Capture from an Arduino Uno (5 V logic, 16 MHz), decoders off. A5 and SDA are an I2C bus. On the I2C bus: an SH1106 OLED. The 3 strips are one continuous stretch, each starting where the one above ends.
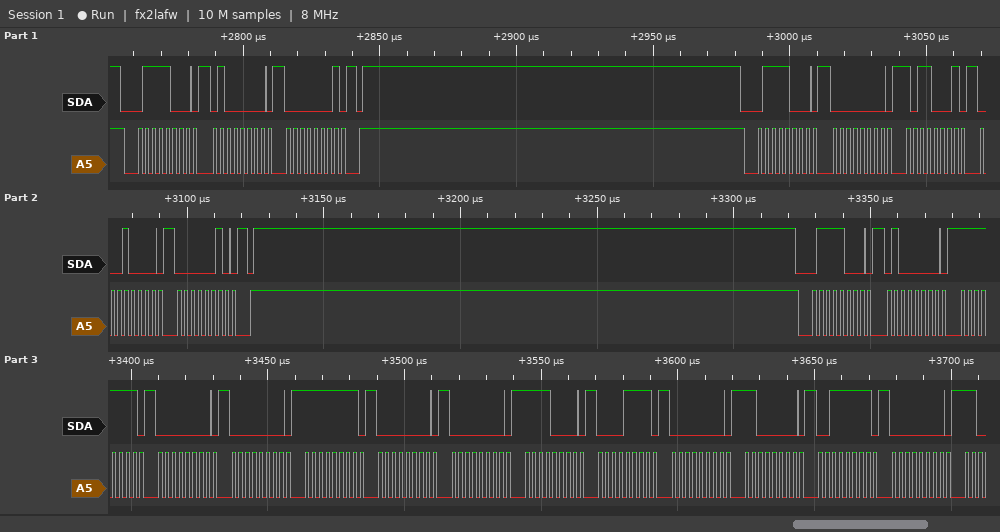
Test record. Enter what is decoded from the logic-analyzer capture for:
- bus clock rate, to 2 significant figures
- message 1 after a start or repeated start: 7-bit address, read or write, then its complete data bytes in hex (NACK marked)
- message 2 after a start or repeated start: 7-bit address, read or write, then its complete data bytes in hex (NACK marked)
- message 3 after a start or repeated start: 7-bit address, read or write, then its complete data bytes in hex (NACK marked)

400 kHz
0x3C write: 40 01
0x3C write: 00 B1 10 02
0x3C write: 40 FF 00 00 FF 00 00 F0 0F 00 C0 3F 00
